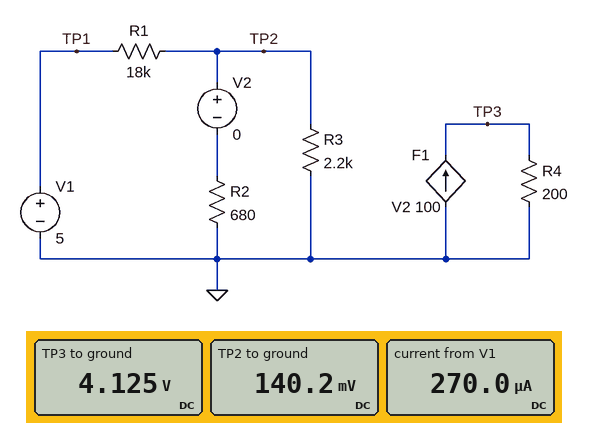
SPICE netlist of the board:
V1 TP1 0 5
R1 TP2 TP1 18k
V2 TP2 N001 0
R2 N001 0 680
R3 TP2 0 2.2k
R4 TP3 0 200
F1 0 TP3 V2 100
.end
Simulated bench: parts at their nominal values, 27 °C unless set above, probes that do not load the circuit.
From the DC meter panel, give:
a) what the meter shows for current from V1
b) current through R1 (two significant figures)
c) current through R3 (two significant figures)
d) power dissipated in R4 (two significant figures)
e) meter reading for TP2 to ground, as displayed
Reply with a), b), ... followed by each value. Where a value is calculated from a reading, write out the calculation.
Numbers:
a) 270.0 µA
b) (5 V - 140.2 mV) / 18 kΩ = 270 µA
c) (140.2 mV) / 2.2 kΩ = 64 µA
d) (4.125 V)^2 / 200 Ω = 85 mW
e) 140.2 mV
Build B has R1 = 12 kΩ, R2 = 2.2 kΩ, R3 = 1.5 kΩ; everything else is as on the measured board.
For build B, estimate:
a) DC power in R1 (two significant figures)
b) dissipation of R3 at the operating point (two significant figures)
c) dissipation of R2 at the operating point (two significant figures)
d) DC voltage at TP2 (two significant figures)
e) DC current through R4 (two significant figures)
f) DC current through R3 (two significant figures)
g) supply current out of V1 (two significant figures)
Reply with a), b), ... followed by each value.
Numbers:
a) 1.8 mW
b) 80 µW
c) 54 µW
d) 350 mV
e) 16 mA
f) 230 µA
g) 390 µA
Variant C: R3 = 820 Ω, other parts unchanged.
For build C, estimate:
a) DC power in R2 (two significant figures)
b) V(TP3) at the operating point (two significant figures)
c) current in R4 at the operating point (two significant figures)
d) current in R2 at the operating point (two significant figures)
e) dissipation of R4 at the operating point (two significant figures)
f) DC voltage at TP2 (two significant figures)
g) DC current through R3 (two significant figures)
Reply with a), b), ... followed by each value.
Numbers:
a) 15 µW
b) 3.0 V
c) 15 mA
d) 150 µA
e) 44 mW
f) 100 mV
g) 120 µA
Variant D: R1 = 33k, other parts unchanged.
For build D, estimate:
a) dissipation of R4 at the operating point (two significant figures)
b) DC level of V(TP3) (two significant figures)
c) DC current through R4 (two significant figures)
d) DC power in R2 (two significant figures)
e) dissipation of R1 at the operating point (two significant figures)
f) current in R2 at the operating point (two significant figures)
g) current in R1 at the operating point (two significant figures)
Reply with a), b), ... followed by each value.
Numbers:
a) 26 mW
b) 2.3 V
c) 11 mA
d) 8.8 µW
e) 730 µW
f) 110 µA
g) 150 µA
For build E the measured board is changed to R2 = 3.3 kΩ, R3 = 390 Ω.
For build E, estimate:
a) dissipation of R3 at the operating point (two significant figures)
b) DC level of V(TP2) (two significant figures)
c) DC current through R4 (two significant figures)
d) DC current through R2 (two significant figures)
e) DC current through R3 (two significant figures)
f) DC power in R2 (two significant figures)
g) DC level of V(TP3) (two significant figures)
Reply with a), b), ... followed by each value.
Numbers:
a) 23 µW
b) 95 mV
c) 2.9 mA
d) 29 µA
e) 240 µA
f) 2.7 µW
g) 580 mV
